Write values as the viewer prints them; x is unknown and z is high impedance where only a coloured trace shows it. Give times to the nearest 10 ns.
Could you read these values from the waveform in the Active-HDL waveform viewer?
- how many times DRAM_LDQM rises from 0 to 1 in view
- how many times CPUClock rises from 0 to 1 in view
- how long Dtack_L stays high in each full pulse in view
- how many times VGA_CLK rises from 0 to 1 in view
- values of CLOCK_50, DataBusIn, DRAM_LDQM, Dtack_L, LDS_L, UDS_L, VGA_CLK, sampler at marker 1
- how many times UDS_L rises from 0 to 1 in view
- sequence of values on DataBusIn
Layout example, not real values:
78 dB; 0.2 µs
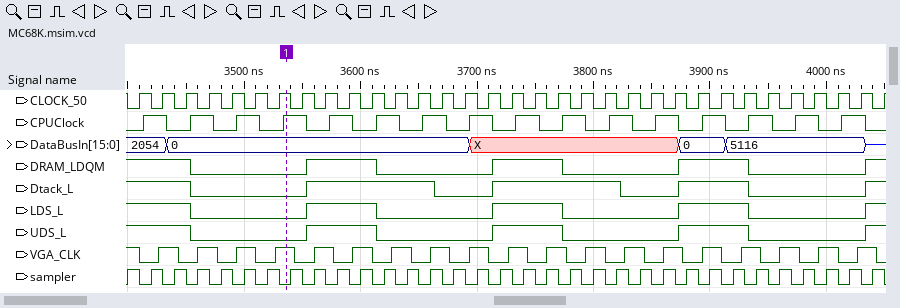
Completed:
4; 16; 110 ns, 110 ns, 60 ns; 19; CLOCK_50=1, DataBusIn=0, DRAM_LDQM=0, Dtack_L=0, LDS_L=0, UDS_L=0, VGA_CLK=1, sampler=0; 4; 2054, 0, X, 0, 5116, z
